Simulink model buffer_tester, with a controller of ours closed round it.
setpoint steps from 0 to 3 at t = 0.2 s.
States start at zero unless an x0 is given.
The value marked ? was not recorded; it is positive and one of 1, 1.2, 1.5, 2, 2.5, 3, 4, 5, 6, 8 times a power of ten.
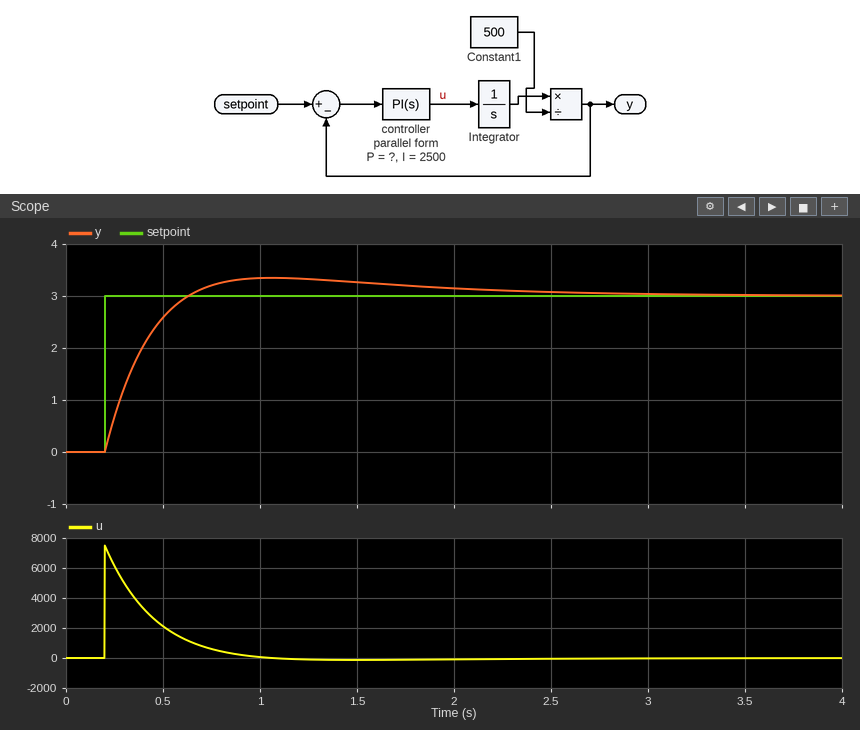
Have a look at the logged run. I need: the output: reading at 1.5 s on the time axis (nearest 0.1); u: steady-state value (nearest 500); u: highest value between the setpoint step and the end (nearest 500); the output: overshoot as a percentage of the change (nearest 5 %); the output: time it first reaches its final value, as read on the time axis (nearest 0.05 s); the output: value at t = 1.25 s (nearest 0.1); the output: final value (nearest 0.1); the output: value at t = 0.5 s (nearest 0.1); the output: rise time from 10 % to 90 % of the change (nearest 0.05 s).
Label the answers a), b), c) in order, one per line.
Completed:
a) 3.3
b) 0
c) 7500
d) 10 %
e) 0.65 s
f) 3.3
g) 3.0
h) 2.6
i) 0.30 s
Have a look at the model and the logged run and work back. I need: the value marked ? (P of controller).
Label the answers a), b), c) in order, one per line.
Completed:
a) 2500
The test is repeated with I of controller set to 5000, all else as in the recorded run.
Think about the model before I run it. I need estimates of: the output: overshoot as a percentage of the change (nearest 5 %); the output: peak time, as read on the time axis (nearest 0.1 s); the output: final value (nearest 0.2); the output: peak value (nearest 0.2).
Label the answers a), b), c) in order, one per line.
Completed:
a) 20 %
b) 0.9 s
c) 3.0
d) 3.6
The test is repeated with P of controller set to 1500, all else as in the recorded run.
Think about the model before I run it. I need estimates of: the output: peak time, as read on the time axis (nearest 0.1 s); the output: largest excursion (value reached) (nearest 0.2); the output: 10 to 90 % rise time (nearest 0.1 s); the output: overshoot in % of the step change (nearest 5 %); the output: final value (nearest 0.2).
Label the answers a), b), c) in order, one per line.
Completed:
a) 1.2 s
b) 3.6
c) 0.4 s
d) 20 %
e) 3.0
